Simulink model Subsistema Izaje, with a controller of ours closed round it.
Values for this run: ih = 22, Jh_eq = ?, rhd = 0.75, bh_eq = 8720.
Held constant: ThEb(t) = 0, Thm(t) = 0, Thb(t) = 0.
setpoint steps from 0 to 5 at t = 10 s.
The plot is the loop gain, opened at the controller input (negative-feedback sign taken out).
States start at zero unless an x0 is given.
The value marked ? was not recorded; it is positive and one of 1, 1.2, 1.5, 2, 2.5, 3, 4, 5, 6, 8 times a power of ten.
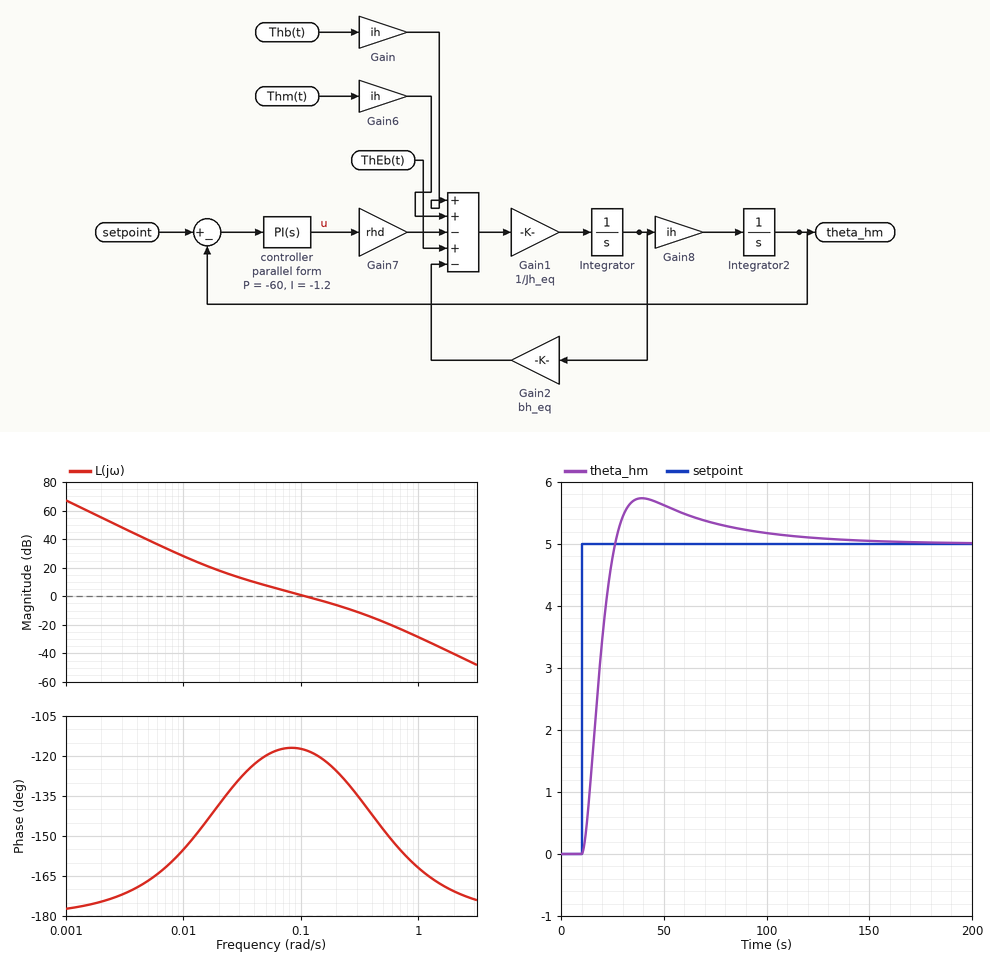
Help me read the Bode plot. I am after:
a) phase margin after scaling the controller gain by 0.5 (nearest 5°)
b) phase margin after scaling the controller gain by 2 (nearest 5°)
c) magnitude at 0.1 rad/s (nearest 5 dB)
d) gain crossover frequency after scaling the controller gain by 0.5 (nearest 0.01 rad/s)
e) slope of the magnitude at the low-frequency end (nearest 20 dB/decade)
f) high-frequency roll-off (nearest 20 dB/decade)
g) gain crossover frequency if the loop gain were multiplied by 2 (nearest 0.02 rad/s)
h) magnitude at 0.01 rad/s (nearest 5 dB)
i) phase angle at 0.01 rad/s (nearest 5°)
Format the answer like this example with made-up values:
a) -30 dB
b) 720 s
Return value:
a) 60°
b) 55°
c) 0 dB
d) 0.06 rad/s
e) -40 dB/decade
f) -40 dB/decade
g) 0.20 rad/s
h) 30 dB
i) -155°
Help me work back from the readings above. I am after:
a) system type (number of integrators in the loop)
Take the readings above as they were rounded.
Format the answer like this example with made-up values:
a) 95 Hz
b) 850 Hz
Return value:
a) 2
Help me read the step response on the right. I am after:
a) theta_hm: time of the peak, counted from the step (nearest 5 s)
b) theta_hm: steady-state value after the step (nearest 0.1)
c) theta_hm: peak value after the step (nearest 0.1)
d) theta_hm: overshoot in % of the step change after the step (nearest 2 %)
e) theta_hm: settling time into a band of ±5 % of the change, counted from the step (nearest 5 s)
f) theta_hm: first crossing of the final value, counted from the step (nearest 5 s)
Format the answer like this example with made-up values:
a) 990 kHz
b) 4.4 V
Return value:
a) 30 s
b) 5.0
c) 5.7
d) 14 %
e) 75 s
f) 15 s
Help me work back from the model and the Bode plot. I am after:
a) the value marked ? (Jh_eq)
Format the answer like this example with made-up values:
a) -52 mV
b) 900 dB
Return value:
a) 25000
